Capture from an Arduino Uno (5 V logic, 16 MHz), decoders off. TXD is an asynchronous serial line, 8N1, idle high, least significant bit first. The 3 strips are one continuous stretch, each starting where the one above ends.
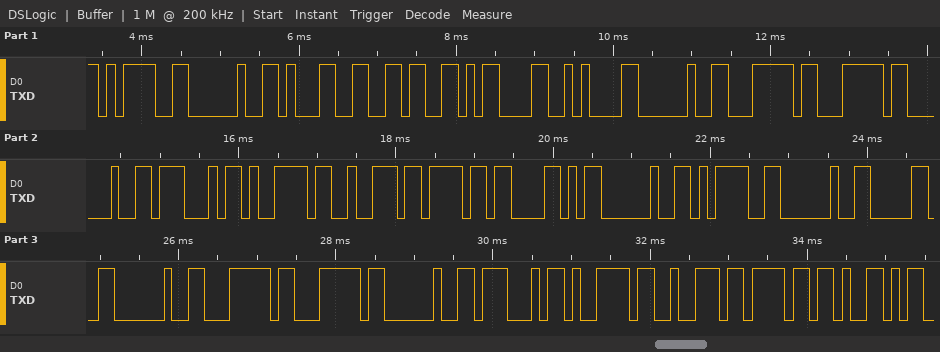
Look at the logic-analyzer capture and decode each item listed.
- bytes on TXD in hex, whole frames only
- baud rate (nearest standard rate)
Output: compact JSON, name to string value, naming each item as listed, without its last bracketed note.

{"bytes on TXD in hex, whole frames only": "3D 20 31 36 0D 0A 20 7C 7C 20 47 79 72 6F 58 20 3D 20 30 20 7C 7C 20 47 79 72 6F 59", "baud rate": "9600 baud"}
